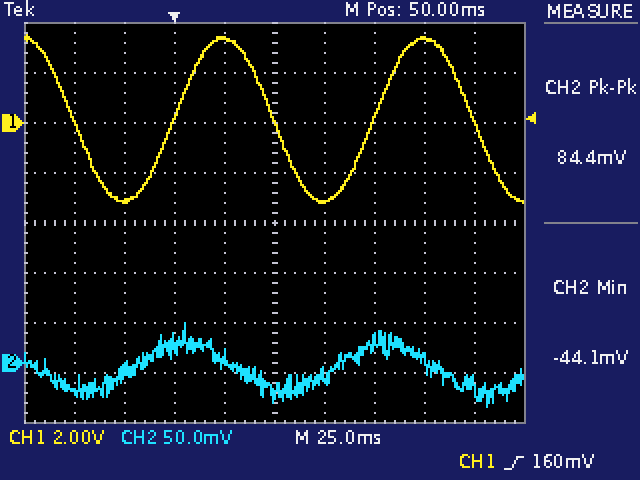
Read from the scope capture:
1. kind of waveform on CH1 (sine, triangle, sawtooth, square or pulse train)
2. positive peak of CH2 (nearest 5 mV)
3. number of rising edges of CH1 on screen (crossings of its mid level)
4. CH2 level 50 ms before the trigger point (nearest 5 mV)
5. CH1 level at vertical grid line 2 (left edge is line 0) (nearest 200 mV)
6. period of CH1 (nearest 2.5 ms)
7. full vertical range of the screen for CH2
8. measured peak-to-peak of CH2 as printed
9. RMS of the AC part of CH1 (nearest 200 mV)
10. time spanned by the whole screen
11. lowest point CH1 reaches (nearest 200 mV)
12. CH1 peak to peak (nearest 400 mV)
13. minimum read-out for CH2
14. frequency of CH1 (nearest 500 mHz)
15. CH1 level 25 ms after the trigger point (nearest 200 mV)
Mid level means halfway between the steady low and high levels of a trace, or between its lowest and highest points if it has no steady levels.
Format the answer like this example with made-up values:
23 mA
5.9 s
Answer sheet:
sine
40 mV
2
-30 mV
-3.2 V
100.0 ms
400 mV
84.4 mV
2.4 V
250 ms
-3.2 V
6.8 V
-44.1 mV
10.0 Hz
3.4 V
